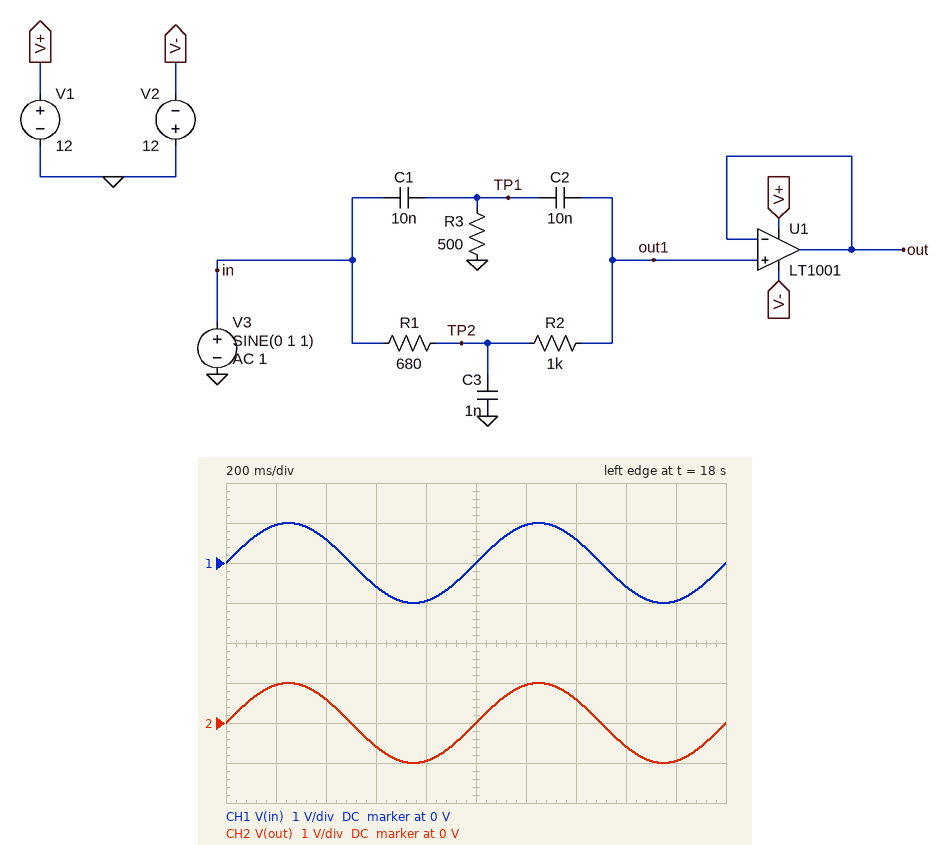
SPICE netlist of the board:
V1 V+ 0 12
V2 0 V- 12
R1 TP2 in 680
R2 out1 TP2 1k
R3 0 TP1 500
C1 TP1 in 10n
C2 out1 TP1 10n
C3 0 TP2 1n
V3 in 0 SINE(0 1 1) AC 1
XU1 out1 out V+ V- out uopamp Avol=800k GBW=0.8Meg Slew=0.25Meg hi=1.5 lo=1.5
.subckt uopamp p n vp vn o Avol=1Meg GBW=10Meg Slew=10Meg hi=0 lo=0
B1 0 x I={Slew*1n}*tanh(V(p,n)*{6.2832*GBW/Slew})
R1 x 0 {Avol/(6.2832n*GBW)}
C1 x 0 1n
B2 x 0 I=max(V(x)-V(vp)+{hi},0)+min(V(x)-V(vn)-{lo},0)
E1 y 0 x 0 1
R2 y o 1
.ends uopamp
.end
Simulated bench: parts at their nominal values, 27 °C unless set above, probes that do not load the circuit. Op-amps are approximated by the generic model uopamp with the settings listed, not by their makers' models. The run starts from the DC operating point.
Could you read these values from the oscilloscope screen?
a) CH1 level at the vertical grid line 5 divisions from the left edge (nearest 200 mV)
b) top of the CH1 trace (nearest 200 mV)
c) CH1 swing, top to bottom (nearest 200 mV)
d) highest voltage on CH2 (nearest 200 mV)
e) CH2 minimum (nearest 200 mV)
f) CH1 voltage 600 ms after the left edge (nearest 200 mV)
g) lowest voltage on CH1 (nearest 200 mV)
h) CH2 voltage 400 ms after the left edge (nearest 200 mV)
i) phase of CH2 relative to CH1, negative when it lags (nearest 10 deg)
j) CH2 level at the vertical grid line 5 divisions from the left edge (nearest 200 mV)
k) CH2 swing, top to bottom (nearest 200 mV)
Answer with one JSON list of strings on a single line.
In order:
["0 V", "1.0 V", "2.0 V", "1.0 V", "-1.0 V", "-600 mV", "-1.0 V", "600 mV", "0 deg", "0 V", "2.0 V"]
